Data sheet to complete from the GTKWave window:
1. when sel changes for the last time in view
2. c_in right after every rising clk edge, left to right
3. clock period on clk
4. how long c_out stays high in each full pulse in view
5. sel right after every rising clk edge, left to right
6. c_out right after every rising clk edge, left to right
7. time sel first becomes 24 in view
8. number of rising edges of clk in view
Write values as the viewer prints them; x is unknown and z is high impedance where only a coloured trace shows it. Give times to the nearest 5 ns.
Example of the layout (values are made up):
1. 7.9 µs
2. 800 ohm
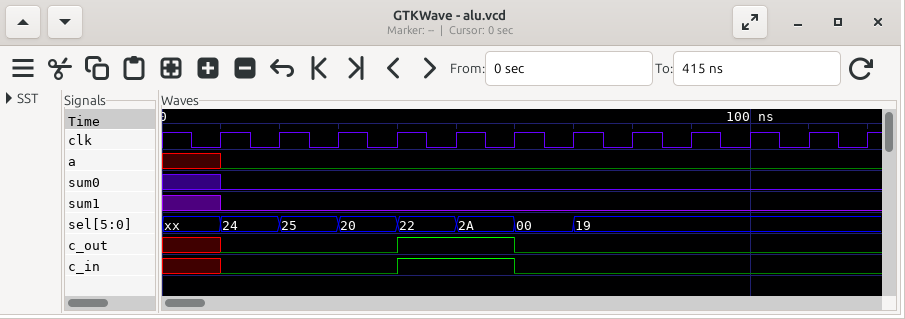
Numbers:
1. 70 ns
2. 0 0 0 1 1 0 0 0 0 0 0 0
3. 10 ns
4. 20 ns
5. 24, 25, 20, 22, 2A, 00, 19, 19, 19, 19, 19, 19
6. 0 0 0 1 1 0 0 0 0 0 0 0
7. 10 ns
8. 12
